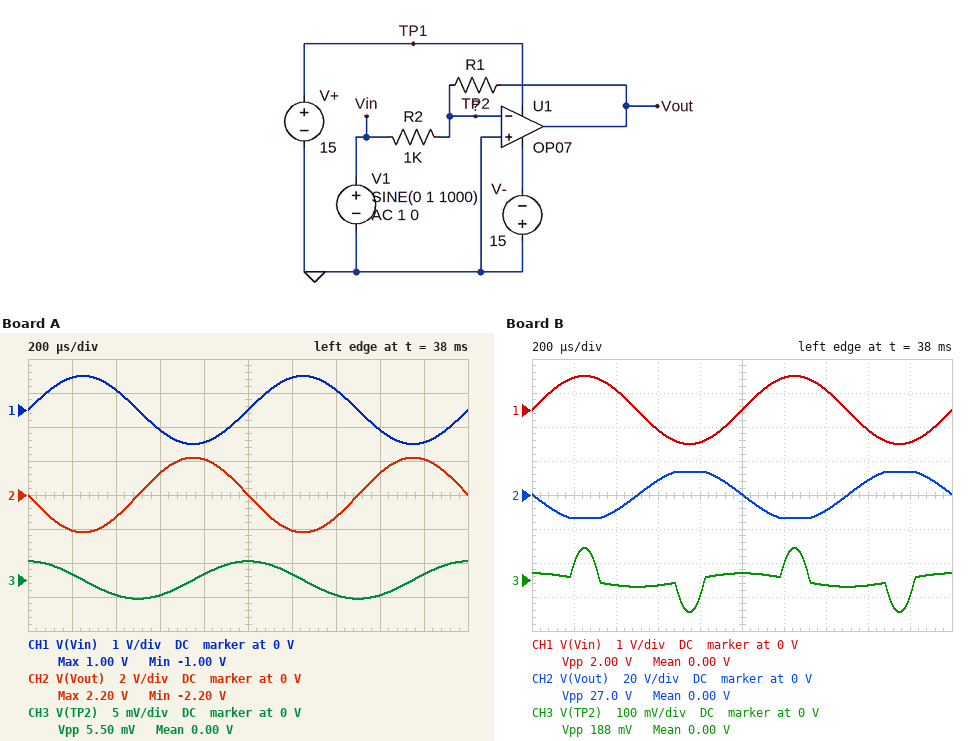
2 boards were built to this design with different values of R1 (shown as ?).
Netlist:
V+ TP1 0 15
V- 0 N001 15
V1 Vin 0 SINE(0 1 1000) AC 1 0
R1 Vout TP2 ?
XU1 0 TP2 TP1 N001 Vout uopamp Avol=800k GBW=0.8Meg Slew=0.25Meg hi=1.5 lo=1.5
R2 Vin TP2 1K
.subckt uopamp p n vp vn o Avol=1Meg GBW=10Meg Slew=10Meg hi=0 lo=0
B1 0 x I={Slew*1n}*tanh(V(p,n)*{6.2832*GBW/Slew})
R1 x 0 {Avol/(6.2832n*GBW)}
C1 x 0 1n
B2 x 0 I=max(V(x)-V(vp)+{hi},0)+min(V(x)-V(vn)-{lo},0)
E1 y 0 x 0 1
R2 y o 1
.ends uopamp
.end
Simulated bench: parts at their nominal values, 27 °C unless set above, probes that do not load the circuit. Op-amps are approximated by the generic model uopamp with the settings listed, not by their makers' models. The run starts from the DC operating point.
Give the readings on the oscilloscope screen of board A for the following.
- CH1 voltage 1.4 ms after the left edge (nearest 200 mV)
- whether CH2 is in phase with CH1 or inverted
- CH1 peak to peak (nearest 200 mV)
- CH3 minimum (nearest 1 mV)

600 mV
inverted
2.0 V
-3 mV
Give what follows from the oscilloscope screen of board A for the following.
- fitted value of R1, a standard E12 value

2.2 kΩ
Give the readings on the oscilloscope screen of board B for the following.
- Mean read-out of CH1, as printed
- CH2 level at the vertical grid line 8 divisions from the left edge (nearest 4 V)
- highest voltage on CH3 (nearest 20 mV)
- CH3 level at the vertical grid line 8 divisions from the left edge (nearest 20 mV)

0.00 V
8 V
100 mV
-20 mV
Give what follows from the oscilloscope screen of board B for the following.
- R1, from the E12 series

15 kΩ
